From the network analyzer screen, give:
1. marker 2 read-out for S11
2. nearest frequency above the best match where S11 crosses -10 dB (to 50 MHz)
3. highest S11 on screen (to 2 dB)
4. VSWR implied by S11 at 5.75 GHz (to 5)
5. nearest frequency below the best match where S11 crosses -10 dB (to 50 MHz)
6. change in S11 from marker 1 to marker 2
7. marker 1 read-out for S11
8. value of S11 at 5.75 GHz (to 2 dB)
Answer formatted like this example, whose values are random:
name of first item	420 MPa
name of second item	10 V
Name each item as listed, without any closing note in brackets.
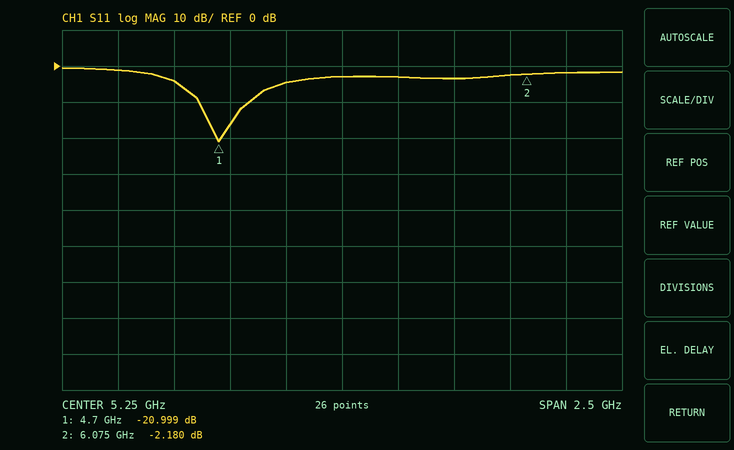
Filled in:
marker 2 read-out for S11	-2.180 dB
nearest frequency above the best match where S11 crosses -10 dB	4.85 GHz
highest S11 on screen	0 dB
VSWR implied by S11 at 5.75 GHz	5
nearest frequency below the best match where S11 crosses -10 dB	4.60 GHz
change in S11 from marker 1 to marker 2	18.819 dB
marker 1 read-out for S11	-20.999 dB
value of S11 at 5.75 GHz	-4 dB
